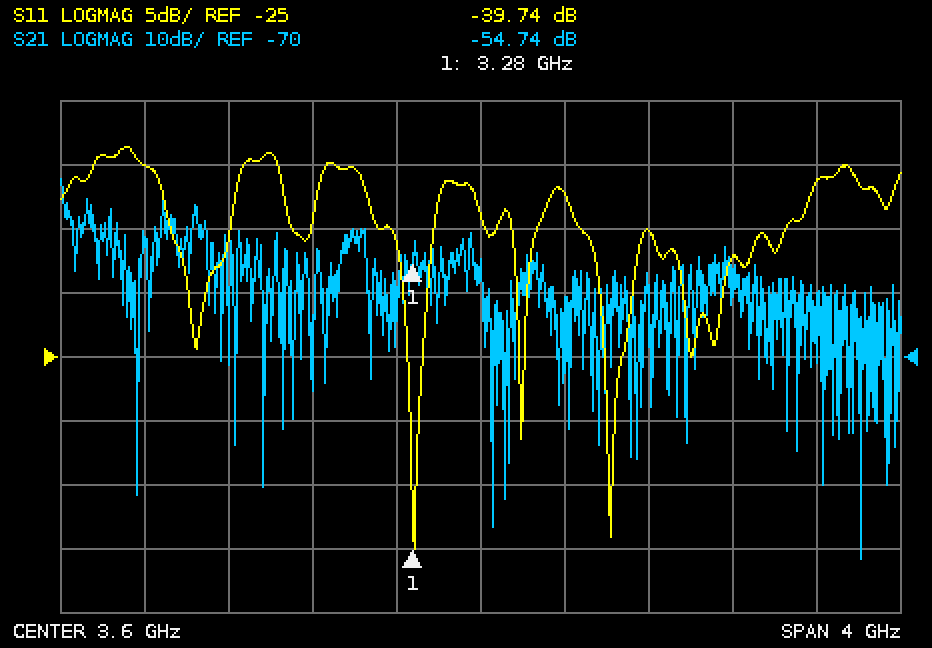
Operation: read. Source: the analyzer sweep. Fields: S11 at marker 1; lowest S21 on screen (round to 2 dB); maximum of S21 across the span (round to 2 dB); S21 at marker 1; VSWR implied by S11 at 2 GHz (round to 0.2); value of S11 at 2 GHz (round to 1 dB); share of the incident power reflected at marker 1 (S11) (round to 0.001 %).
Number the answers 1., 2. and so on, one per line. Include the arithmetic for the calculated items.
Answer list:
1. -39.74 dB
2. -102 dB
3. -42 dB
4. -54.74 dB
5. |Γ| = 10^(-10/20) = 0.3162; VSWR = (1 + 0.3162)/(1 − 0.3162) ≈ 1.92, so 2.0 to the nearest 0.2
6. -10 dB
7. 10^(-39.74/10) ≈ 0.011 %
